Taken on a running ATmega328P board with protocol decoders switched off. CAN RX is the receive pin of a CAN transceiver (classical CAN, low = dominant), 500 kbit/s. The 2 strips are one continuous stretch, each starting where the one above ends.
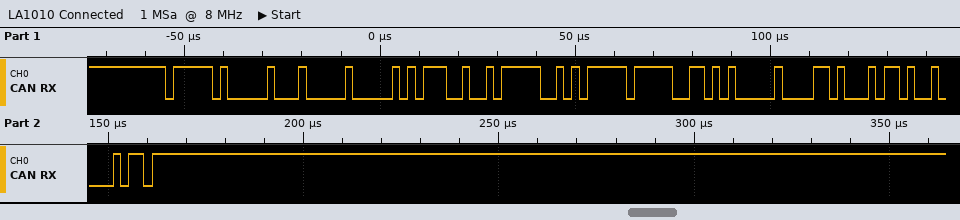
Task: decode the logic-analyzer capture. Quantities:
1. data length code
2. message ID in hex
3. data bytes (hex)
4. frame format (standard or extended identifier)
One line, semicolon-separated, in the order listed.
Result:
8; 0x7E0; 00 B9 2F AB FF 6A 00 D1; standard
